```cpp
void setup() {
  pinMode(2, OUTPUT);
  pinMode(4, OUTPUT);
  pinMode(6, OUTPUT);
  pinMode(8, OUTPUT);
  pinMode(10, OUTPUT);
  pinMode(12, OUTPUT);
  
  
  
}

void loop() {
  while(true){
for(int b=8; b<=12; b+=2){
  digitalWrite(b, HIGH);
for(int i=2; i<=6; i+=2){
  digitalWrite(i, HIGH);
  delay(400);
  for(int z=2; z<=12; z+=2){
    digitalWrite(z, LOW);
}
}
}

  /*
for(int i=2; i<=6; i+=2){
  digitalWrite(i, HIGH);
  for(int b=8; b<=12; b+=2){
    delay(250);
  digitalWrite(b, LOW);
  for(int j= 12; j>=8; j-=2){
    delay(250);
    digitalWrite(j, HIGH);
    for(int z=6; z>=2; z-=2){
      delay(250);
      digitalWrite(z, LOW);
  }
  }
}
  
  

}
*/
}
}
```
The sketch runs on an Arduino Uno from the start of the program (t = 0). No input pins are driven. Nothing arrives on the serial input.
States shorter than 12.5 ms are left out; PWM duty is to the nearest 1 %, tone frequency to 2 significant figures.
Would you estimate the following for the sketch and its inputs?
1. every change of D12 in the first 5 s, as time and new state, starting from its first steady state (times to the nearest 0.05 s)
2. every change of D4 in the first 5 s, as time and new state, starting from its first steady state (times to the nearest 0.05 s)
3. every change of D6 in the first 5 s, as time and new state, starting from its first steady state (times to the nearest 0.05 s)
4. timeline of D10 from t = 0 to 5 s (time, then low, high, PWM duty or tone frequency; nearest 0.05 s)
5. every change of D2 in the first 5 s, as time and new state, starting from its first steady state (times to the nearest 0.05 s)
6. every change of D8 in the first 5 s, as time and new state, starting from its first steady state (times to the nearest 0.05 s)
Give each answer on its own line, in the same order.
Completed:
0 s low; 2.4 s high; 2.8 s low
0 s low; 0.4 s high; 0.8 s low; 1.6 s high; 2 s low; 2.8 s high; 3.2 s low; 4 s high; 4.4 s low
0 s low; 0.8 s high; 1.2 s low; 2 s high; 2.4 s low; 3.2 s high; 3.6 s low; 4.4 s high; 4.8 s low
0 s low; 1.2 s high; 1.6 s low; 4.8 s high
0 s high; 0.4 s low; 1.2 s high; 1.6 s low; 2.4 s high; 2.8 s low; 3.6 s high; 4 s low; 4.8 s high
0 s high; 0.4 s low; 3.6 s high; 4 s low
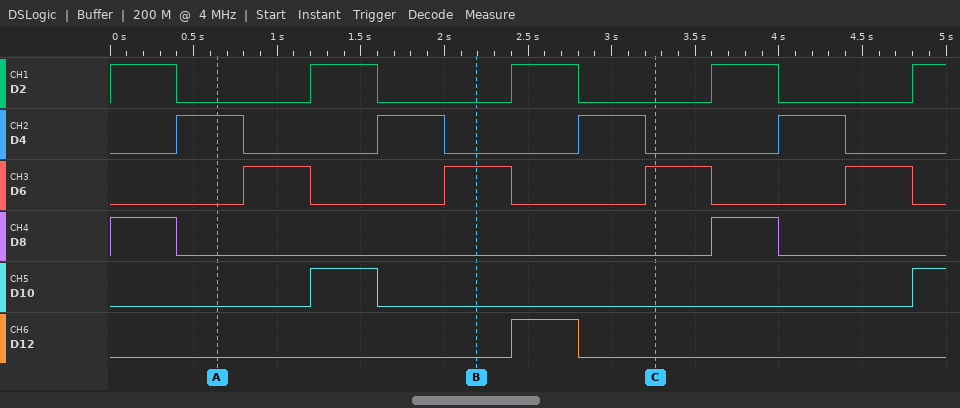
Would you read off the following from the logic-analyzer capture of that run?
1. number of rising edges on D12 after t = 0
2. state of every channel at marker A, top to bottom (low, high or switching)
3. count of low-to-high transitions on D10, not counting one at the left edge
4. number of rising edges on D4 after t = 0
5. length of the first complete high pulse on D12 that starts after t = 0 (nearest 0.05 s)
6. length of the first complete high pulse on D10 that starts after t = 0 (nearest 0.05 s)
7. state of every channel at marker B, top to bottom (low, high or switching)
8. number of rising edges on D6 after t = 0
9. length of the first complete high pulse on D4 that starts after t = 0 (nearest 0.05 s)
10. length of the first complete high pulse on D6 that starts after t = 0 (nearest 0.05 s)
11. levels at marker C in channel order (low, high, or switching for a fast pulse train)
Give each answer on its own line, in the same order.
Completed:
1
D2 low, D4 high, D6 low, D8 low, D10 low, D12 low
2
4
0.40 s
0.40 s
D2 low, D4 low, D6 high, D8 low, D10 low, D12 low
4
0.40 s
0.40 s
D2 low, D4 low, D6 high, D8 low, D10 low, D12 low
